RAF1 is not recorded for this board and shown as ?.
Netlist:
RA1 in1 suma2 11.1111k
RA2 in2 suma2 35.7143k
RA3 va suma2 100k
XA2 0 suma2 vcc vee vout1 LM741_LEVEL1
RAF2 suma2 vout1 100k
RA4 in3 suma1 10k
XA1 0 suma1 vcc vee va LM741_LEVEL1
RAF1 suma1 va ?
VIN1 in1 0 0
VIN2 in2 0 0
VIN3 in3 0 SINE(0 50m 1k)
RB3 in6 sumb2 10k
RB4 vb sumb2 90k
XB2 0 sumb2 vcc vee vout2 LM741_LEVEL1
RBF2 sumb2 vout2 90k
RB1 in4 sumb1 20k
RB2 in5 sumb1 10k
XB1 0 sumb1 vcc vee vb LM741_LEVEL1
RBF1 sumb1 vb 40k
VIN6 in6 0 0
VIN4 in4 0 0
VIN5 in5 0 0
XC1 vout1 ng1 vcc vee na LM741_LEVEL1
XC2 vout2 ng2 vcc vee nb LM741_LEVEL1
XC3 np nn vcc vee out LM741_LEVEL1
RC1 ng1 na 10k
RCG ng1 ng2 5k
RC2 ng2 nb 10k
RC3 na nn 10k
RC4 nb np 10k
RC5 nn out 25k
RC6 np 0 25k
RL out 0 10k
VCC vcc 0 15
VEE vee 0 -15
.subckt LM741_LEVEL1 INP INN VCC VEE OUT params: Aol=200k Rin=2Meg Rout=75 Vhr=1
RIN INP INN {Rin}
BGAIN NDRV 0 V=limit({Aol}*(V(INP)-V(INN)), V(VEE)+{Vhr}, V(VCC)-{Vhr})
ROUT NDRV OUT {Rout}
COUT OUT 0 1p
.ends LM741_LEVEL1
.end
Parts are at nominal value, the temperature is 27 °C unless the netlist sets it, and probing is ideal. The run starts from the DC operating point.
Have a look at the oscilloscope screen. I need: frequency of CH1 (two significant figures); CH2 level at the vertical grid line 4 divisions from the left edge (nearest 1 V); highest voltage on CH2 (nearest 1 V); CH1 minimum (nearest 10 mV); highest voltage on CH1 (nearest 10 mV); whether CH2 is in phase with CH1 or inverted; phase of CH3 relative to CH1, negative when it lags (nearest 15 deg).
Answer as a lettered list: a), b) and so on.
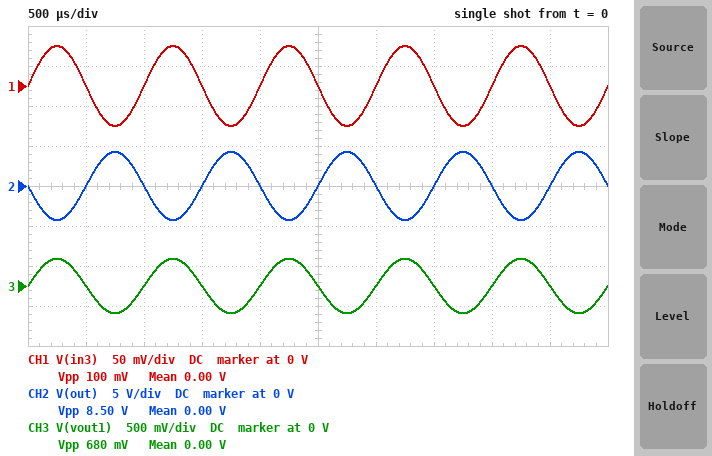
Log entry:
a) 1.0 kHz
b) 0 V
c) 4 V
d) -50 mV
e) 50 mV
f) inverted
g) 0 deg
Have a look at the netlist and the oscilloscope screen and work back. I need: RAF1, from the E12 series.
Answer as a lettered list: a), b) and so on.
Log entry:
a) 68 kΩ
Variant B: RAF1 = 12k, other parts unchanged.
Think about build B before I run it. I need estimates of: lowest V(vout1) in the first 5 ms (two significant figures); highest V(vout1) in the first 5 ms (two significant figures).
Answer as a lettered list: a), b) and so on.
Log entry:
a) -60 mV
b) 60 mV
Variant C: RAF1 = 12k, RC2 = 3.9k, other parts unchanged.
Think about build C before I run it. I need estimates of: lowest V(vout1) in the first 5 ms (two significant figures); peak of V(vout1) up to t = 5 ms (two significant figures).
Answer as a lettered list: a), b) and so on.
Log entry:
a) -60 mV
b) 60 mV
